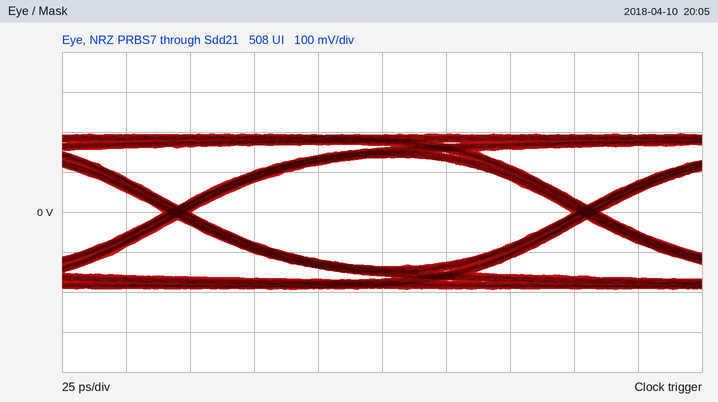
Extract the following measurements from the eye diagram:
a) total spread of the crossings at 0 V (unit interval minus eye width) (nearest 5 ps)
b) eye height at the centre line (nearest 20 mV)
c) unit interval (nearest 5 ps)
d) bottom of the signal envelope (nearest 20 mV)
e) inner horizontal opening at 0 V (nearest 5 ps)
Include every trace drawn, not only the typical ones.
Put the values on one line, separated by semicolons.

10 ps; 280 mV; 160 ps; -200 mV; 150 ps
